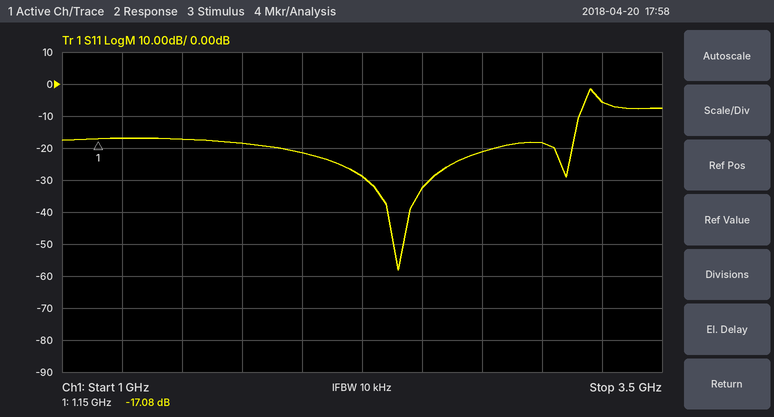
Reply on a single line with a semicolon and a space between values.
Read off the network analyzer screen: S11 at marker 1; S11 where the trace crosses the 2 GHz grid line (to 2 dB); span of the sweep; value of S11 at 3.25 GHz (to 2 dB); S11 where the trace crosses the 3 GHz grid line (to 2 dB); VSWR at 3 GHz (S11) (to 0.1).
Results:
-17.08 dB; -22 dB; 2.5 GHz; -6 dB; -18 dB; 1.3
